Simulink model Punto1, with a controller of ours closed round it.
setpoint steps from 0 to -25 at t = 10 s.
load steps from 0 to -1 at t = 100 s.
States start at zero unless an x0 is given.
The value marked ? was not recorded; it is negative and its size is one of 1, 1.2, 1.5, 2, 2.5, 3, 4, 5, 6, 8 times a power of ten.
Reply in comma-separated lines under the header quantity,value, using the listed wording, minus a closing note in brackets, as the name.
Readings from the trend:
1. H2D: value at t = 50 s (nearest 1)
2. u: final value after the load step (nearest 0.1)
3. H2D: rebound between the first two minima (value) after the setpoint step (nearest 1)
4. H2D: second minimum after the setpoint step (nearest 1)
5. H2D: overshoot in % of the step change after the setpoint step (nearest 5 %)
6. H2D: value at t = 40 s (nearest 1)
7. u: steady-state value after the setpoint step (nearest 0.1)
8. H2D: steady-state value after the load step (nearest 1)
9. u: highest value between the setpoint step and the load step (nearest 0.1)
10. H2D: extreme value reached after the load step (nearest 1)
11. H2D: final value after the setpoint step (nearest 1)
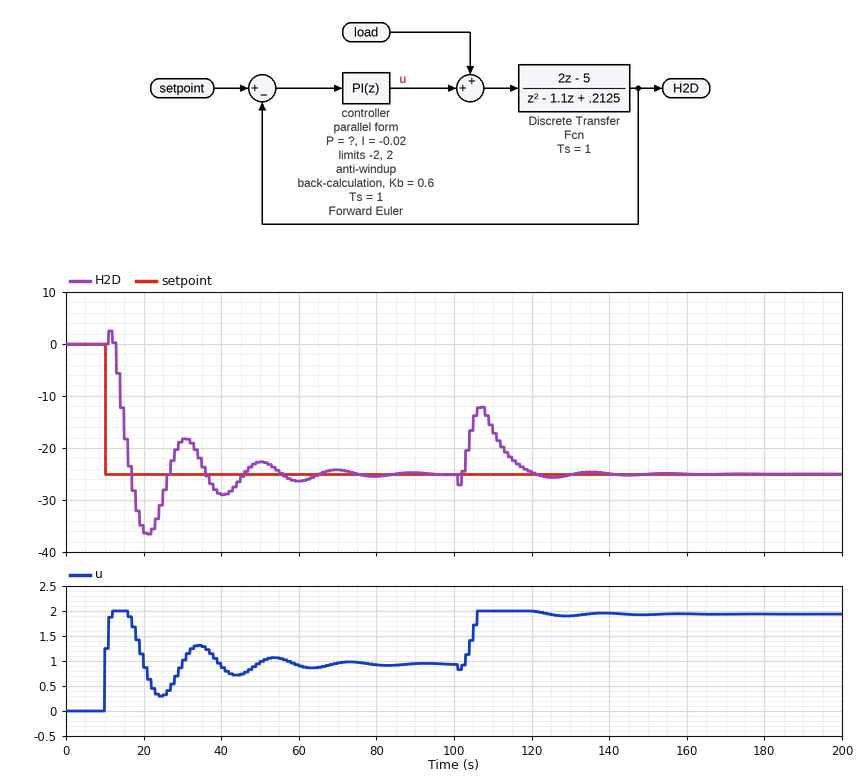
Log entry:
quantity,value
H2D: value at t = 50 s,-23
u: final value after the load step,1.9
H2D: rebound between the first two minima (value) after the setpoint step,-18
H2D: second minimum after the setpoint step,-29
H2D: overshoot in % of the step change after the setpoint step,45 %
H2D: value at t = 40 s,-29
u: steady-state value after the setpoint step,0.9
H2D: steady-state value after the load step,-25
u: highest value between the setpoint step and the load step,2.0
H2D: extreme value reached after the load step,-12
H2D: final value after the setpoint step,-25
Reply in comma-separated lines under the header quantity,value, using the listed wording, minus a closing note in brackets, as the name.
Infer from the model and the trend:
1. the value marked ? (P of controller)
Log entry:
quantity,value
the value marked ?,-0.05
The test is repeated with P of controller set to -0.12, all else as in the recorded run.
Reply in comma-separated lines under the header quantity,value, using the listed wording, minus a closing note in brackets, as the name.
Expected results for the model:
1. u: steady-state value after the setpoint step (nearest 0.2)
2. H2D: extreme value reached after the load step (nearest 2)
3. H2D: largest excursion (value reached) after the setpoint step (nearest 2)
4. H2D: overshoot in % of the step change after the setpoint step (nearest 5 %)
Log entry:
quantity,value
u: steady-state value after the setpoint step,1.0
H2D: extreme value reached after the load step,-14
H2D: largest excursion (value reached) after the setpoint step,-28
H2D: overshoot in % of the step change after the setpoint step,10 %
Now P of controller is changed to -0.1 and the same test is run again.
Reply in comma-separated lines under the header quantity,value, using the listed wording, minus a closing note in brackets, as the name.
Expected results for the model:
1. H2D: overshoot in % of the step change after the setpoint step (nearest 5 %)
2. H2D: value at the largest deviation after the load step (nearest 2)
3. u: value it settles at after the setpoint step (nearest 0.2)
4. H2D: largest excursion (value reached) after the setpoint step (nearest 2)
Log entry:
quantity,value
H2D: overshoot in % of the step change after the setpoint step,15 %
H2D: value at the largest deviation after the load step,-14
u: value it settles at after the setpoint step,1.0
H2D: largest excursion (value reached) after the setpoint step,-28
